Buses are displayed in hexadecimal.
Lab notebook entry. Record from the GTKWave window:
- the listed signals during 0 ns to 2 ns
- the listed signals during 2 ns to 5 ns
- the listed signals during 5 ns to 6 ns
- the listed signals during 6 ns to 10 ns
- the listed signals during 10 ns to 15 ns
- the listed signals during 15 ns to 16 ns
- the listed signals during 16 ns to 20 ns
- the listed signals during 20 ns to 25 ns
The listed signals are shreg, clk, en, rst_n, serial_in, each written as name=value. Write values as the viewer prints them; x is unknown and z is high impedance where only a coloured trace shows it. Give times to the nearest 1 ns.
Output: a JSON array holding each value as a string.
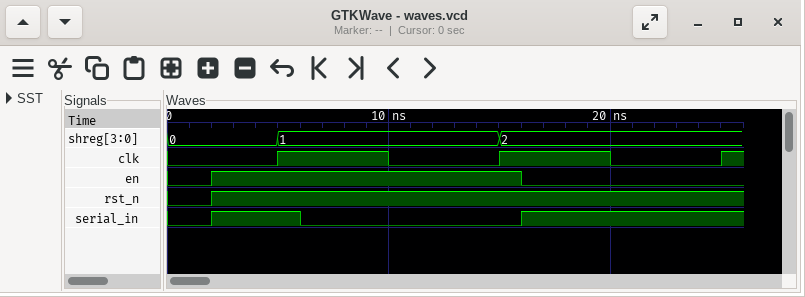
["shreg=0, clk=0, en=0, rst_n=0, serial_in=0", "shreg=0, clk=0, en=1, rst_n=1, serial_in=1", "shreg=1, clk=1, en=1, rst_n=1, serial_in=1", "shreg=1, clk=1, en=1, rst_n=1, serial_in=0", "shreg=1, clk=0, en=1, rst_n=1, serial_in=0", "shreg=2, clk=1, en=1, rst_n=1, serial_in=0", "shreg=2, clk=1, en=0, rst_n=1, serial_in=1", "shreg=2, clk=0, en=0, rst_n=1, serial_in=1"]
